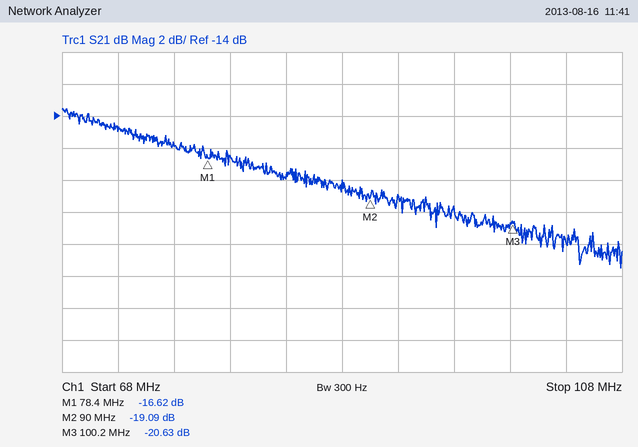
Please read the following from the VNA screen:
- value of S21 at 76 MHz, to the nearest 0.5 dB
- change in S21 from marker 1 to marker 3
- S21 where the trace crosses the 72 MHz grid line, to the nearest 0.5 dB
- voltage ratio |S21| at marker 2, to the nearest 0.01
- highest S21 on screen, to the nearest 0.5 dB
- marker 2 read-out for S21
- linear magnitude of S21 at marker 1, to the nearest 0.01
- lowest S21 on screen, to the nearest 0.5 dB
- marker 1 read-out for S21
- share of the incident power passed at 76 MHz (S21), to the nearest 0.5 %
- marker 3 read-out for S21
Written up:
-16.0 dB
-4.01 dB
-15.0 dB
0.11
-13.5 dB
-19.09 dB
0.15
-23.5 dB
-16.62 dB
2.5 %
-20.63 dB
